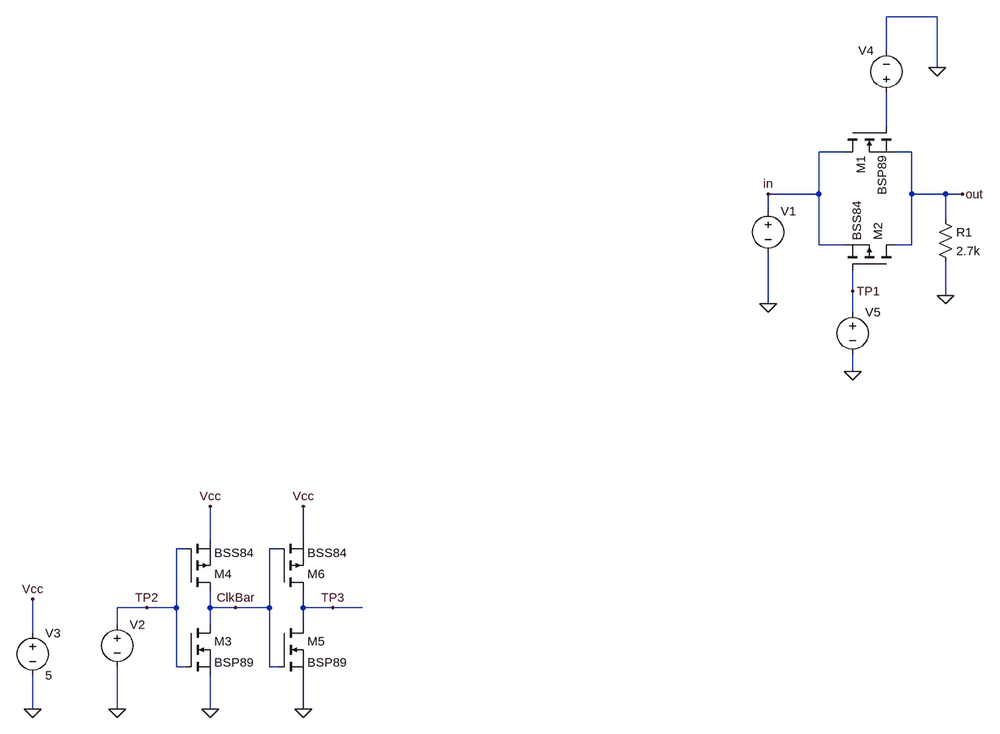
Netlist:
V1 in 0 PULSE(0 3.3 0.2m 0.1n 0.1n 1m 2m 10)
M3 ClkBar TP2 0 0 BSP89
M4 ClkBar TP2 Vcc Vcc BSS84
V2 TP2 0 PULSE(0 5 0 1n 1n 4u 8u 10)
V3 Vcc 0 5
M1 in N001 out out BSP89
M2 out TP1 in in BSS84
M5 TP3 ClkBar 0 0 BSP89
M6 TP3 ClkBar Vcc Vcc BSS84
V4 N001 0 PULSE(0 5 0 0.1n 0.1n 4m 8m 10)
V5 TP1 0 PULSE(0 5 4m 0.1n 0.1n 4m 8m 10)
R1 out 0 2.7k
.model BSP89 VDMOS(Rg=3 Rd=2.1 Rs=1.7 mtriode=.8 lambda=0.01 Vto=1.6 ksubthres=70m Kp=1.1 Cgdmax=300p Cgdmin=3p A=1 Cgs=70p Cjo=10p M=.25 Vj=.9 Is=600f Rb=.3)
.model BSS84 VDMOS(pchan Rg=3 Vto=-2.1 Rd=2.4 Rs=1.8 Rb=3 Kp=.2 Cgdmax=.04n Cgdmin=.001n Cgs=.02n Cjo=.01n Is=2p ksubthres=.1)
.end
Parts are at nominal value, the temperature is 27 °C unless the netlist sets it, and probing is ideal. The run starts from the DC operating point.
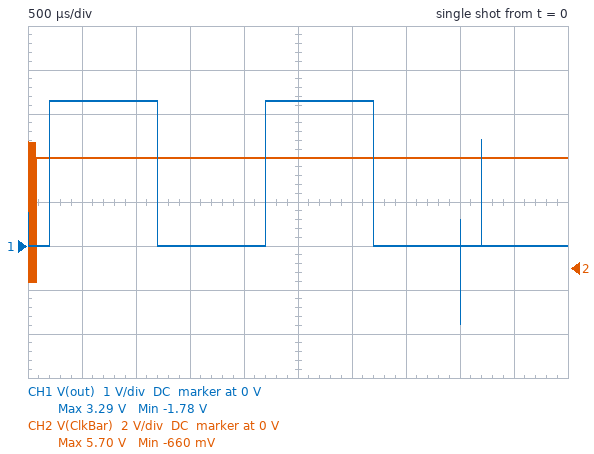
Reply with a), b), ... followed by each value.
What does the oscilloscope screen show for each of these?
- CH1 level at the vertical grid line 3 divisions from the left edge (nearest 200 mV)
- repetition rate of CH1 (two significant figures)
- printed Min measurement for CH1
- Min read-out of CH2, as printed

a) 0 V
b) 500 Hz
c) -1.78 V
d) -660 mV
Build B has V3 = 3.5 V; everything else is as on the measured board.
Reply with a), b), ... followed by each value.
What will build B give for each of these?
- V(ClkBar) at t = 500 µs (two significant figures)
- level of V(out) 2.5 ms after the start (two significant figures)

a) 3.5 V
b) 3.3 V
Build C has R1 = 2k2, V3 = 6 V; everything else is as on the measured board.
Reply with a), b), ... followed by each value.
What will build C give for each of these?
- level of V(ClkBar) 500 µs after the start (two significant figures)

a) 6.0 V
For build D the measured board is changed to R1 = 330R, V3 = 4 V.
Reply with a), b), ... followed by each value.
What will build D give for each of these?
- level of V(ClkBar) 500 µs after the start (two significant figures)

a) 4.0 V
